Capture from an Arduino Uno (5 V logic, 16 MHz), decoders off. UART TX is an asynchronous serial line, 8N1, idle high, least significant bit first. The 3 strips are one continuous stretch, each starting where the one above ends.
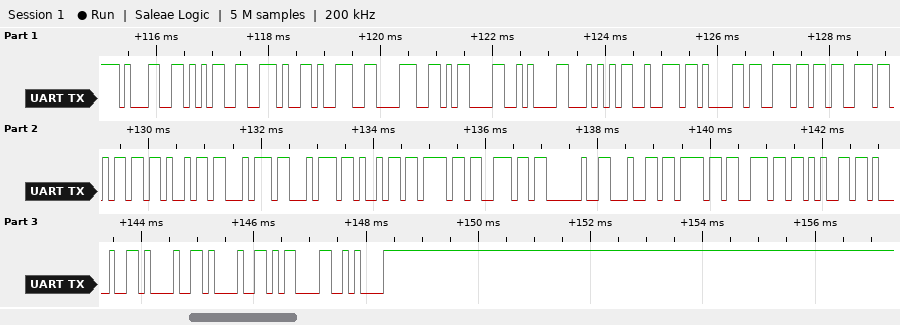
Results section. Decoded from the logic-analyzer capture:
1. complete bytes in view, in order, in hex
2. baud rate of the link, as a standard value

31 35 2E 39 38 0D 0A 54 72 61 6E 73 6D 69 74 74 69 6F 6E 20 64 6F 6E 65 21 21 21 0D 0A
9600 baud
